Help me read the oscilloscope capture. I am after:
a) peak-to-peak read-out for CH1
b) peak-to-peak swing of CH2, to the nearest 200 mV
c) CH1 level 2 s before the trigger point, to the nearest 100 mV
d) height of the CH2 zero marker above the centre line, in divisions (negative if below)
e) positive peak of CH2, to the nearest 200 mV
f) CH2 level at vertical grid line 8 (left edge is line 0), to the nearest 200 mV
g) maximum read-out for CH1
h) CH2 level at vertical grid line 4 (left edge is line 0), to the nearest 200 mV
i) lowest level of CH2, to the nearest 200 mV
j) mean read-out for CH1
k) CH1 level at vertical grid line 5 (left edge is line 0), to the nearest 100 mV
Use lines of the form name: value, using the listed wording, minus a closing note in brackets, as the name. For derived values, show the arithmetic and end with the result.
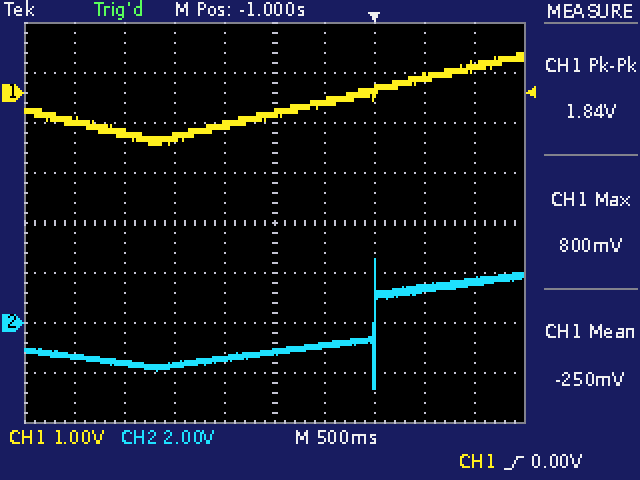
peak-to-peak read-out for CH1: 1.84 V
peak-to-peak swing of CH2, to the nearest 200 mV: 2.6 V − (-2.6 V) = 5.2 V
CH1 level 2 s before the trigger point, to the nearest 100 mV: -900 mV
height of the CH2 zero marker above the centre line, in divisions: -2.0 div
positive peak of CH2, to the nearest 200 mV: 2.6 V
CH2 level at vertical grid line 8 (left edge is line 0), to the nearest 200 mV: 1.4 V
maximum read-out for CH1: 800 mV
CH2 level at vertical grid line 4 (left edge is line 0), to the nearest 200 mV: -1.4 V
lowest level of CH2, to the nearest 200 mV: -2.6 V
mean read-out for CH1: -250 mV
CH1 level at vertical grid line 5 (left edge is line 0), to the nearest 100 mV: -400 mV
